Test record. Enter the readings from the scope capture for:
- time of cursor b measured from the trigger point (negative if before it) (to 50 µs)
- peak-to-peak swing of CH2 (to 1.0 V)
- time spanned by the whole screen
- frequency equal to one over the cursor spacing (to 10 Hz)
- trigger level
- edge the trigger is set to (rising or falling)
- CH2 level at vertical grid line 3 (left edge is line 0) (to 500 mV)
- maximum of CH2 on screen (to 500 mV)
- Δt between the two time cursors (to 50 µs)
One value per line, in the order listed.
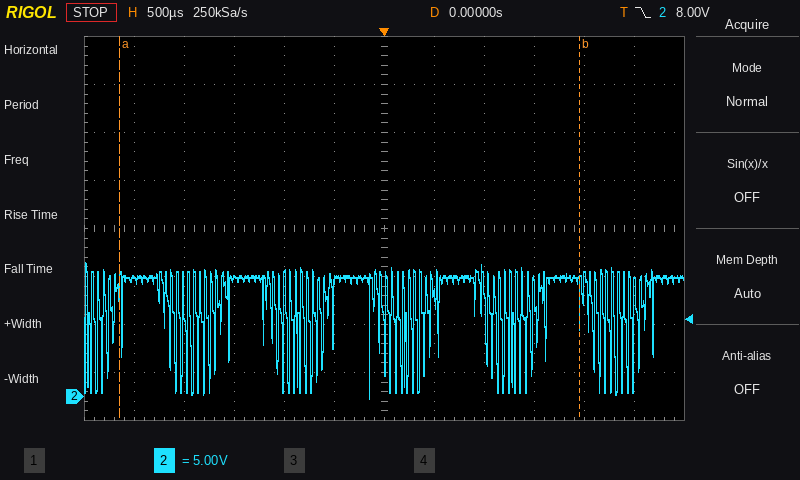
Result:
+1.95 ms
14.0 V
6 ms
220 Hz
8.00 V
falling
12.5 V
14.0 V
4.60 ms
